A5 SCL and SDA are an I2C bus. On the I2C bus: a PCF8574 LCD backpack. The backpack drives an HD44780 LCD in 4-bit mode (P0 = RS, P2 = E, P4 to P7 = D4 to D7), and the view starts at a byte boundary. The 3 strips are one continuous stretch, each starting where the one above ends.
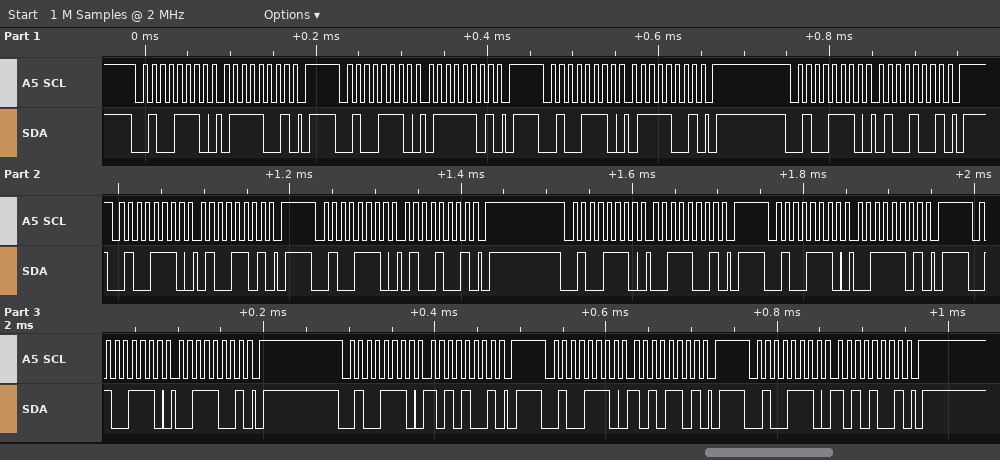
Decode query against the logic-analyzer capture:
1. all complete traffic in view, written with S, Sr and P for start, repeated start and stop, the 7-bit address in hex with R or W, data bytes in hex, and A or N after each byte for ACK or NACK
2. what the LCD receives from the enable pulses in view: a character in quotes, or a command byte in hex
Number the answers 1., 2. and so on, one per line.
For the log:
1. S 27W A 79 A P S 27W A 7D A P S 27W A 79 A P S 27W A 49 A P S 27W A 4D A P S 27W A 49 A P S 27W A 39 A P S 27W A 3D A P S 27W A 39 A P S 27W A A9 A P S 27W A AD A P S 27W A A9 A P
2. 't' ':'
